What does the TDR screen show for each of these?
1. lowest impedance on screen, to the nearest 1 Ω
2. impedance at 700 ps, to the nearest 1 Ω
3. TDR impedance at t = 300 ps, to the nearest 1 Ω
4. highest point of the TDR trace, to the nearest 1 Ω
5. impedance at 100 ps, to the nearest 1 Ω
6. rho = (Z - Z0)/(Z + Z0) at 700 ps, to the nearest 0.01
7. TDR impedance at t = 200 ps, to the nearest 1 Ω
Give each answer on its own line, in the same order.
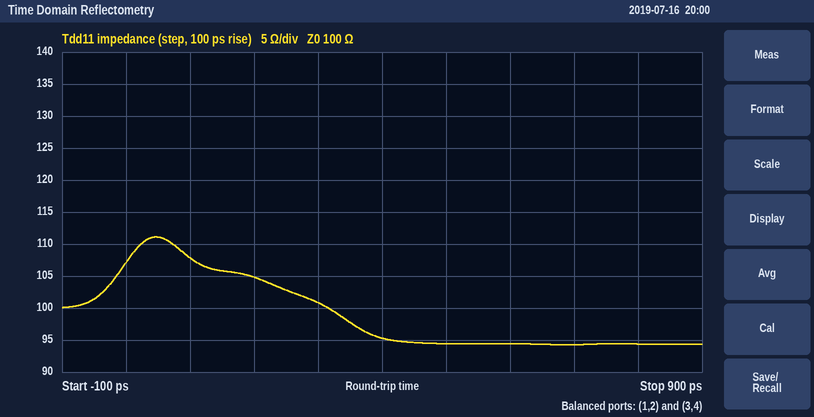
94 Ω
94 Ω
101 Ω
111 Ω
108 Ω
-0.03
105 Ω
